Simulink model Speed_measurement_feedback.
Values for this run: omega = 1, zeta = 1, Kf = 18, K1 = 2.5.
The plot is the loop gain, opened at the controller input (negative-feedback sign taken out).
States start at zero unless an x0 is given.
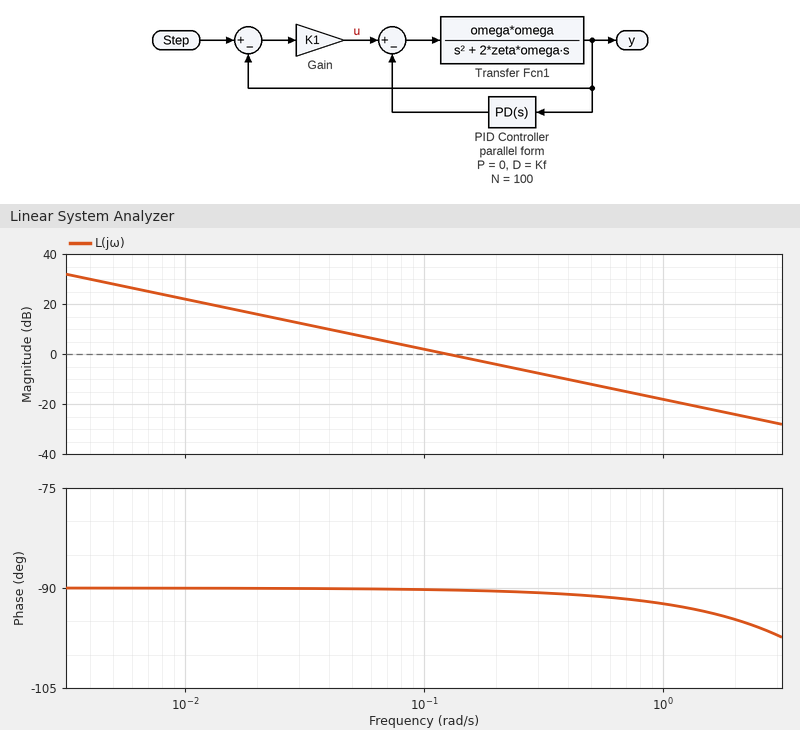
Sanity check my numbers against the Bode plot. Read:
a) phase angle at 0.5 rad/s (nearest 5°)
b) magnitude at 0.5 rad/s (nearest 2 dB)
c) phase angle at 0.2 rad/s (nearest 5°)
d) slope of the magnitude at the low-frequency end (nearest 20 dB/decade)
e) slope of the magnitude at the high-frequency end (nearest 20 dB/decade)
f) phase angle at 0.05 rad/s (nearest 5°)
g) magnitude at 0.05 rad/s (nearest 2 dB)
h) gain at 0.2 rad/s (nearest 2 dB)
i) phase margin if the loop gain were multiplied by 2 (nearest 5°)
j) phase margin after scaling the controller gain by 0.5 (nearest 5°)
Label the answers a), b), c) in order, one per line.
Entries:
a) -90°
b) -12 dB
c) -90°
d) -20 dB/decade
e) -20 dB/decade
f) -90°
g) 8 dB
h) -4 dB
i) 90°
j) 90°
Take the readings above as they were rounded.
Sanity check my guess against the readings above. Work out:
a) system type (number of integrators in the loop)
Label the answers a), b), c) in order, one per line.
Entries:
a) 1
